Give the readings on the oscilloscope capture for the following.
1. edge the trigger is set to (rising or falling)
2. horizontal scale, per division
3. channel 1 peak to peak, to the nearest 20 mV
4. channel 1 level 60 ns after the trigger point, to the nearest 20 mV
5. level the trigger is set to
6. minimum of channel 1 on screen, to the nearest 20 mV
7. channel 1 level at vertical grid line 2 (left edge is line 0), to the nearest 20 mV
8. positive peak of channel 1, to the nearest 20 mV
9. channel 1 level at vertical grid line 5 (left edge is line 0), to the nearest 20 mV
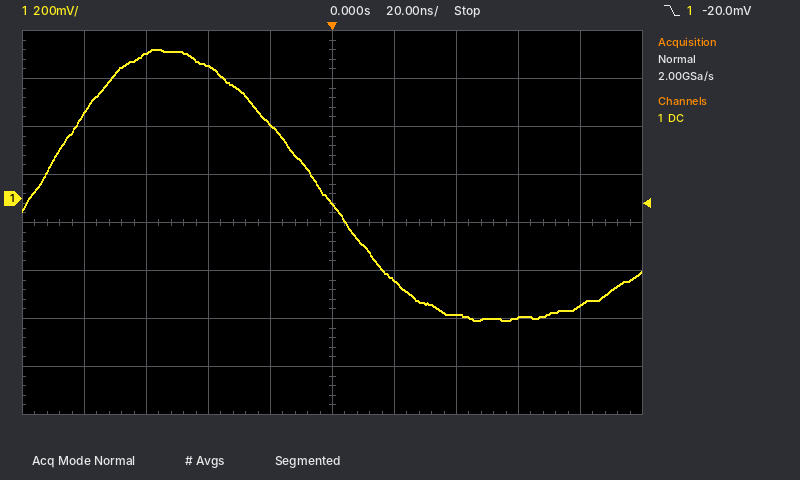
falling
20 ns
1.12 V
-500 mV
-20.0 mV
-500 mV
600 mV
620 mV
-20 mV
